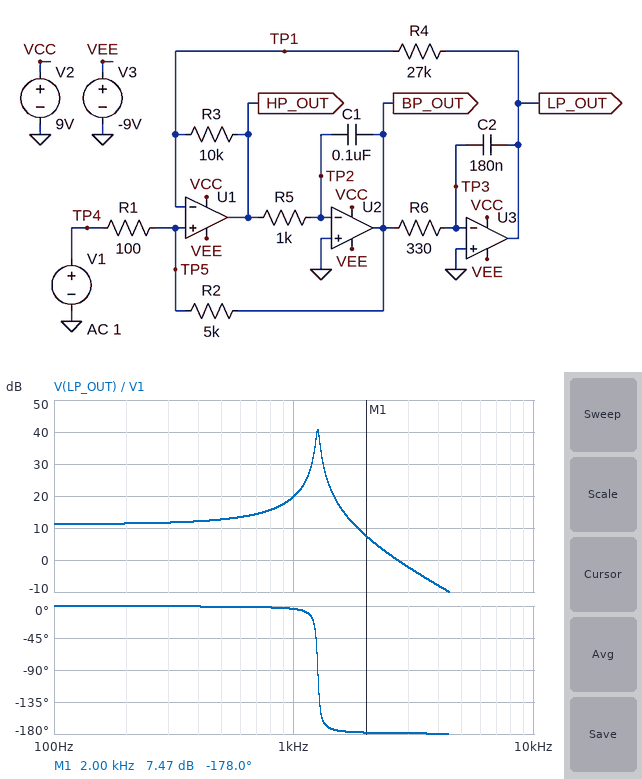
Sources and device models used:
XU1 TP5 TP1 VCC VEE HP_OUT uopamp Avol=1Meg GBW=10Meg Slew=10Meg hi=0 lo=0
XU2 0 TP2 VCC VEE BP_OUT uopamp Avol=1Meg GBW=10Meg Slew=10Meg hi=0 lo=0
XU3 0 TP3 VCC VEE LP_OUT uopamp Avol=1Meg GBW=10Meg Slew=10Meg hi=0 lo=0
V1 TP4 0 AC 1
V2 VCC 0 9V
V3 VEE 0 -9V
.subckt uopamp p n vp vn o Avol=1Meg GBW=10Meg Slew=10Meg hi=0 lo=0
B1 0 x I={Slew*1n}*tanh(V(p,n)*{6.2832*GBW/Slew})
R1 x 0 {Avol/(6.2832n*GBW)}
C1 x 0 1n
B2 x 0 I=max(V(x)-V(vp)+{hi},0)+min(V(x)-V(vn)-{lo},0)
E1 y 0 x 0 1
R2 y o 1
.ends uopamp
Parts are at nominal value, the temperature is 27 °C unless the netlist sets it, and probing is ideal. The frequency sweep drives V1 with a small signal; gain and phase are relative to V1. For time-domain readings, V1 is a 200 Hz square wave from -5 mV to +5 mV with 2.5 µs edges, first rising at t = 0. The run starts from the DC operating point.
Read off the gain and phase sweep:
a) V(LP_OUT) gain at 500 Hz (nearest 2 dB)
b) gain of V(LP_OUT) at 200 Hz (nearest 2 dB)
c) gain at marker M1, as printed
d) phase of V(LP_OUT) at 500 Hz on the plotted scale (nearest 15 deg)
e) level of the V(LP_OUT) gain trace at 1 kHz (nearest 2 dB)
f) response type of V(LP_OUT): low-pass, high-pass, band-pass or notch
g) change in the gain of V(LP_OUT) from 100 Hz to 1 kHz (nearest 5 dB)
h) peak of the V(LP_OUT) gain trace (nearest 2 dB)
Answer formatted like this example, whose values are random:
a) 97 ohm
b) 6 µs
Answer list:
a) 12 dB
b) 12 dB
c) 7.47 dB
d) 0 deg
e) 20 dB
f) low-pass
g) 10 dB
h) 40 dB
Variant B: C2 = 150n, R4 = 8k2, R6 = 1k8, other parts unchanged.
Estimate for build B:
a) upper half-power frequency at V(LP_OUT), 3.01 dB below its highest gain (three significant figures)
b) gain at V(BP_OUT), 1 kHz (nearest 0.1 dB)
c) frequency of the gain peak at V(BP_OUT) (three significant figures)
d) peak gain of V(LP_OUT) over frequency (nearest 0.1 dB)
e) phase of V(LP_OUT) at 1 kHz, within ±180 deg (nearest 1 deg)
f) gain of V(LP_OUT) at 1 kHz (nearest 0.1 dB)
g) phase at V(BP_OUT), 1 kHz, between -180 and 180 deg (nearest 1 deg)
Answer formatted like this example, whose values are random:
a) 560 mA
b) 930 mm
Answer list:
a) 1.10 kHz
b) 26.7 dB
c) 1.07 kHz
d) 28.9 dB
e) -26 deg
f) 22.1 dB
g) -116 deg
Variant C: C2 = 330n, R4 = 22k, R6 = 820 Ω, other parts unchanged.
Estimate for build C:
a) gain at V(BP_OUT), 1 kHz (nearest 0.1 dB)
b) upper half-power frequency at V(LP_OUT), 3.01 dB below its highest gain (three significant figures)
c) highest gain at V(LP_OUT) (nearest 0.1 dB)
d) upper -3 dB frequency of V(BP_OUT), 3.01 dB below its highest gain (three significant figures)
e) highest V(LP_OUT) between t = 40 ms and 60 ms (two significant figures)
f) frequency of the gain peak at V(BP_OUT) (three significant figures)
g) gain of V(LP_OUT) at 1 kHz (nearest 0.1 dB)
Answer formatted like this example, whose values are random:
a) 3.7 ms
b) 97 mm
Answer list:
a) 11.9 dB
b) 674 Hz
c) 33.1 dB
d) 675 Hz
e) 56 mV
f) 652 Hz
g) 7.3 dB
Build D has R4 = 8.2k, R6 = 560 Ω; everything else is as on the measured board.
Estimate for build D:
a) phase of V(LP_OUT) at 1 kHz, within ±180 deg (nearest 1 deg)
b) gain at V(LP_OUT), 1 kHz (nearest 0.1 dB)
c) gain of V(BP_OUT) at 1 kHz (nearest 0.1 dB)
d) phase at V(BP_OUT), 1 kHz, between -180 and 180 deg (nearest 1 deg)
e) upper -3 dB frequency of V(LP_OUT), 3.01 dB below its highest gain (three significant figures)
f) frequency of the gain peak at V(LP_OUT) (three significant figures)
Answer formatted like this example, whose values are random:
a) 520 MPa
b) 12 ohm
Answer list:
a) -2 deg
b) 8.5 dB
c) 4.5 dB
d) -92 deg
e) 1.78 kHz
f) 1.75 kHz
